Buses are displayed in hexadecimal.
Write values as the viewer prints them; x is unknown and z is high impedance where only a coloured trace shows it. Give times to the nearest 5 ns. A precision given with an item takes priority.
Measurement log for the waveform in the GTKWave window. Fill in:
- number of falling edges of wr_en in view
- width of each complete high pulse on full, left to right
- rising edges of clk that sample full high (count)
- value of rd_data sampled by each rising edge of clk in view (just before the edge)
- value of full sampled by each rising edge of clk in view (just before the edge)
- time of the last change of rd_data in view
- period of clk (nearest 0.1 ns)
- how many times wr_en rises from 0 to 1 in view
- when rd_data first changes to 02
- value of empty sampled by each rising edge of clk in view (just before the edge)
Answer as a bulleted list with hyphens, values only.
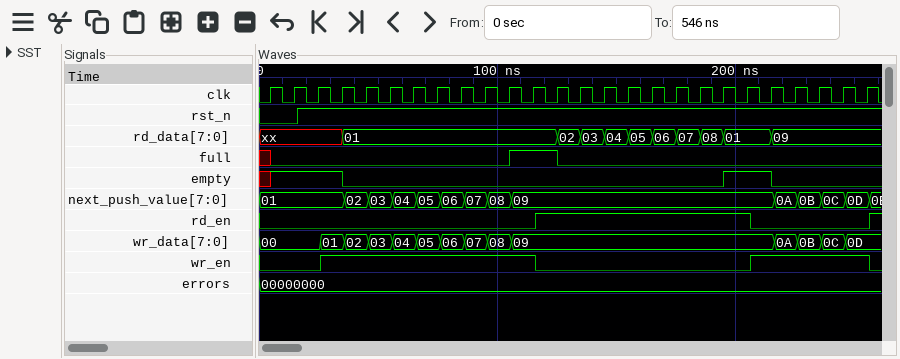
- 2
- 20 ns
- 2
- xx, xx, xx, xx, 01, 01, 01, 01, 01, 01, 01, 01, 01, 02, 03, 04, 05, 06, 07, 08, 01, 01, 09, 09, 09, 09
- x 0 0 0 0 0 0 0 0 0 0 1 1 0 0 0 0 0 0 0 0 0 0 0 0 0
- 215 ns
- 10 ns
- 2
- 125 ns
- x 1 1 1 0 0 0 0 0 0 0 0 0 0 0 0 0 0 0 0 1 1 0 0 0 0
